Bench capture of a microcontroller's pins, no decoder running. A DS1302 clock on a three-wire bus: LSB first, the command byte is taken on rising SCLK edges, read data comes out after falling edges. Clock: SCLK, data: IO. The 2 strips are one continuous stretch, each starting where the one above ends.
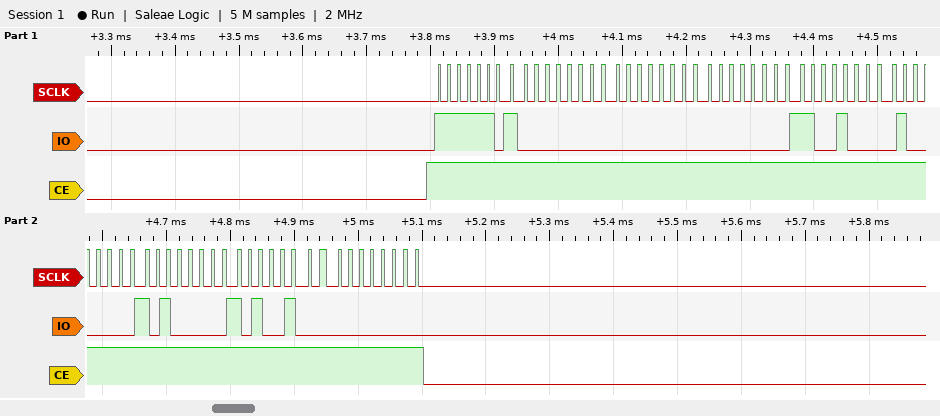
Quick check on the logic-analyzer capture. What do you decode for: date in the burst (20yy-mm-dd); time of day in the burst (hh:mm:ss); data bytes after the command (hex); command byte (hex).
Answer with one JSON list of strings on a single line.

["2025-02-13", "00:00:00", "00 00 00 13 02 05 25 00", "0xBF"]
